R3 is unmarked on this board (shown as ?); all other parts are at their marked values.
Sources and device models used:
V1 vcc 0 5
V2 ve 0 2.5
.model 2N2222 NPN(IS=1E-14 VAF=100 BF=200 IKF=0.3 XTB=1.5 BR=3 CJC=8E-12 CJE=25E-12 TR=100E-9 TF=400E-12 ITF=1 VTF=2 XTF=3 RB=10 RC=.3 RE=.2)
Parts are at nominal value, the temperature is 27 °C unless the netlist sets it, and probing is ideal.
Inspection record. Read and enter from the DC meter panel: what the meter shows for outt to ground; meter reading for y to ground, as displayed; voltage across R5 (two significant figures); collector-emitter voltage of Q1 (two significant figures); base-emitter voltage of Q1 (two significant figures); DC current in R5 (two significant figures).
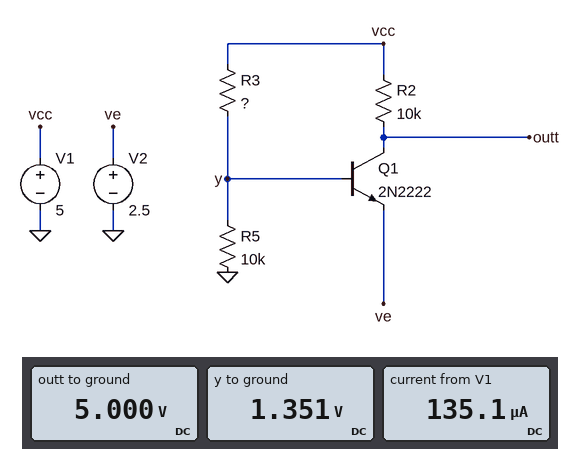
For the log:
5.000 V
1.351 V
1.4 V
2.5 V
-1.1 V
140 µA
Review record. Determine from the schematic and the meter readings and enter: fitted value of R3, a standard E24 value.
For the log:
27 kΩ
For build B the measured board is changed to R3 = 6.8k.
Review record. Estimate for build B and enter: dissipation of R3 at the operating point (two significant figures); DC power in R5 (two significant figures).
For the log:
600 µW
890 µW
